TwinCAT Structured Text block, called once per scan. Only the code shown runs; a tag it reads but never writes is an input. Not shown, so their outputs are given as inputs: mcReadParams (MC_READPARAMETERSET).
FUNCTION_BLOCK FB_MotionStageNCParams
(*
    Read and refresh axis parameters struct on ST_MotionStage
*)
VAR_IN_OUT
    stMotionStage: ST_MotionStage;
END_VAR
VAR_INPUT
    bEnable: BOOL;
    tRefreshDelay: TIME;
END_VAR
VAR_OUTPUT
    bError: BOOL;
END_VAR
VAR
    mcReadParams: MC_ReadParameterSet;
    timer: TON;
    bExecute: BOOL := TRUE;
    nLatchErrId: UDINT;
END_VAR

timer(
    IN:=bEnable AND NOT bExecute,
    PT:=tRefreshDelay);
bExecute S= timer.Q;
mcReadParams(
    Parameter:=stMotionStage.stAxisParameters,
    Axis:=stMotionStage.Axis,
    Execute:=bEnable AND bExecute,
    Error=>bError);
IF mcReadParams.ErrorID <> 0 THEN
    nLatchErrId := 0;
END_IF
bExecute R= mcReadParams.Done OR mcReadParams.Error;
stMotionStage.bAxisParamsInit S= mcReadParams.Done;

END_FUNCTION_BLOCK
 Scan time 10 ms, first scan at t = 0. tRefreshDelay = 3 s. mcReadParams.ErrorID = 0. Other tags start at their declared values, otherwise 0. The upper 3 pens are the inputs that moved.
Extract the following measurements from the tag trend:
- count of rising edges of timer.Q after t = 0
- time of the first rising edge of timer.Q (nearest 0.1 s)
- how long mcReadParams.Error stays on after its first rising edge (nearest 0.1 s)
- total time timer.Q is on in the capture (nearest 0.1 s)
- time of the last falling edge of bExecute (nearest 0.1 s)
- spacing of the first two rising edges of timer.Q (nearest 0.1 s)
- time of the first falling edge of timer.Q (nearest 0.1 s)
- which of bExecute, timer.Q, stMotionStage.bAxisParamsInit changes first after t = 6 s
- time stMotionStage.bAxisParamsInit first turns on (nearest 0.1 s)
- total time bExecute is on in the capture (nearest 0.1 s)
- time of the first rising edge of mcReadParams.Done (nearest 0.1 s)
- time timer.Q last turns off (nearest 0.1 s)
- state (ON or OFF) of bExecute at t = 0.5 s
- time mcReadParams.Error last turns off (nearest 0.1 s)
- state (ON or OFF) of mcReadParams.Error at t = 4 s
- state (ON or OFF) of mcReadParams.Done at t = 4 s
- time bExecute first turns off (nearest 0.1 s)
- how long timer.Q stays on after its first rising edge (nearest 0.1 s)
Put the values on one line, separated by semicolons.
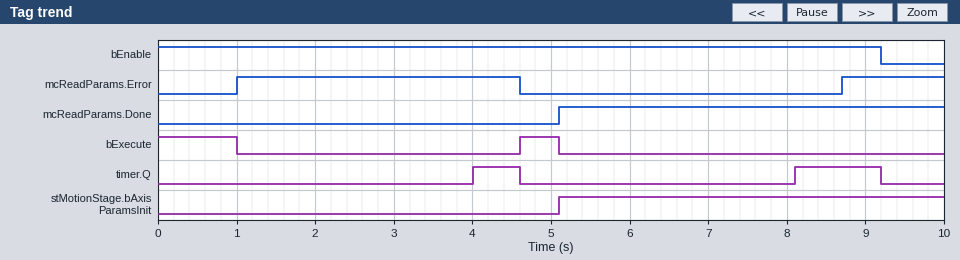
2; 4.0 s; 3.6 s; 1.7 s; 5.1 s; 4.1 s; 4.6 s; timer.Q; 5.1 s; 1.5 s; 5.1 s; 9.2 s; ON; 4.6 s; ON; OFF; 1.0 s; 0.6 s
